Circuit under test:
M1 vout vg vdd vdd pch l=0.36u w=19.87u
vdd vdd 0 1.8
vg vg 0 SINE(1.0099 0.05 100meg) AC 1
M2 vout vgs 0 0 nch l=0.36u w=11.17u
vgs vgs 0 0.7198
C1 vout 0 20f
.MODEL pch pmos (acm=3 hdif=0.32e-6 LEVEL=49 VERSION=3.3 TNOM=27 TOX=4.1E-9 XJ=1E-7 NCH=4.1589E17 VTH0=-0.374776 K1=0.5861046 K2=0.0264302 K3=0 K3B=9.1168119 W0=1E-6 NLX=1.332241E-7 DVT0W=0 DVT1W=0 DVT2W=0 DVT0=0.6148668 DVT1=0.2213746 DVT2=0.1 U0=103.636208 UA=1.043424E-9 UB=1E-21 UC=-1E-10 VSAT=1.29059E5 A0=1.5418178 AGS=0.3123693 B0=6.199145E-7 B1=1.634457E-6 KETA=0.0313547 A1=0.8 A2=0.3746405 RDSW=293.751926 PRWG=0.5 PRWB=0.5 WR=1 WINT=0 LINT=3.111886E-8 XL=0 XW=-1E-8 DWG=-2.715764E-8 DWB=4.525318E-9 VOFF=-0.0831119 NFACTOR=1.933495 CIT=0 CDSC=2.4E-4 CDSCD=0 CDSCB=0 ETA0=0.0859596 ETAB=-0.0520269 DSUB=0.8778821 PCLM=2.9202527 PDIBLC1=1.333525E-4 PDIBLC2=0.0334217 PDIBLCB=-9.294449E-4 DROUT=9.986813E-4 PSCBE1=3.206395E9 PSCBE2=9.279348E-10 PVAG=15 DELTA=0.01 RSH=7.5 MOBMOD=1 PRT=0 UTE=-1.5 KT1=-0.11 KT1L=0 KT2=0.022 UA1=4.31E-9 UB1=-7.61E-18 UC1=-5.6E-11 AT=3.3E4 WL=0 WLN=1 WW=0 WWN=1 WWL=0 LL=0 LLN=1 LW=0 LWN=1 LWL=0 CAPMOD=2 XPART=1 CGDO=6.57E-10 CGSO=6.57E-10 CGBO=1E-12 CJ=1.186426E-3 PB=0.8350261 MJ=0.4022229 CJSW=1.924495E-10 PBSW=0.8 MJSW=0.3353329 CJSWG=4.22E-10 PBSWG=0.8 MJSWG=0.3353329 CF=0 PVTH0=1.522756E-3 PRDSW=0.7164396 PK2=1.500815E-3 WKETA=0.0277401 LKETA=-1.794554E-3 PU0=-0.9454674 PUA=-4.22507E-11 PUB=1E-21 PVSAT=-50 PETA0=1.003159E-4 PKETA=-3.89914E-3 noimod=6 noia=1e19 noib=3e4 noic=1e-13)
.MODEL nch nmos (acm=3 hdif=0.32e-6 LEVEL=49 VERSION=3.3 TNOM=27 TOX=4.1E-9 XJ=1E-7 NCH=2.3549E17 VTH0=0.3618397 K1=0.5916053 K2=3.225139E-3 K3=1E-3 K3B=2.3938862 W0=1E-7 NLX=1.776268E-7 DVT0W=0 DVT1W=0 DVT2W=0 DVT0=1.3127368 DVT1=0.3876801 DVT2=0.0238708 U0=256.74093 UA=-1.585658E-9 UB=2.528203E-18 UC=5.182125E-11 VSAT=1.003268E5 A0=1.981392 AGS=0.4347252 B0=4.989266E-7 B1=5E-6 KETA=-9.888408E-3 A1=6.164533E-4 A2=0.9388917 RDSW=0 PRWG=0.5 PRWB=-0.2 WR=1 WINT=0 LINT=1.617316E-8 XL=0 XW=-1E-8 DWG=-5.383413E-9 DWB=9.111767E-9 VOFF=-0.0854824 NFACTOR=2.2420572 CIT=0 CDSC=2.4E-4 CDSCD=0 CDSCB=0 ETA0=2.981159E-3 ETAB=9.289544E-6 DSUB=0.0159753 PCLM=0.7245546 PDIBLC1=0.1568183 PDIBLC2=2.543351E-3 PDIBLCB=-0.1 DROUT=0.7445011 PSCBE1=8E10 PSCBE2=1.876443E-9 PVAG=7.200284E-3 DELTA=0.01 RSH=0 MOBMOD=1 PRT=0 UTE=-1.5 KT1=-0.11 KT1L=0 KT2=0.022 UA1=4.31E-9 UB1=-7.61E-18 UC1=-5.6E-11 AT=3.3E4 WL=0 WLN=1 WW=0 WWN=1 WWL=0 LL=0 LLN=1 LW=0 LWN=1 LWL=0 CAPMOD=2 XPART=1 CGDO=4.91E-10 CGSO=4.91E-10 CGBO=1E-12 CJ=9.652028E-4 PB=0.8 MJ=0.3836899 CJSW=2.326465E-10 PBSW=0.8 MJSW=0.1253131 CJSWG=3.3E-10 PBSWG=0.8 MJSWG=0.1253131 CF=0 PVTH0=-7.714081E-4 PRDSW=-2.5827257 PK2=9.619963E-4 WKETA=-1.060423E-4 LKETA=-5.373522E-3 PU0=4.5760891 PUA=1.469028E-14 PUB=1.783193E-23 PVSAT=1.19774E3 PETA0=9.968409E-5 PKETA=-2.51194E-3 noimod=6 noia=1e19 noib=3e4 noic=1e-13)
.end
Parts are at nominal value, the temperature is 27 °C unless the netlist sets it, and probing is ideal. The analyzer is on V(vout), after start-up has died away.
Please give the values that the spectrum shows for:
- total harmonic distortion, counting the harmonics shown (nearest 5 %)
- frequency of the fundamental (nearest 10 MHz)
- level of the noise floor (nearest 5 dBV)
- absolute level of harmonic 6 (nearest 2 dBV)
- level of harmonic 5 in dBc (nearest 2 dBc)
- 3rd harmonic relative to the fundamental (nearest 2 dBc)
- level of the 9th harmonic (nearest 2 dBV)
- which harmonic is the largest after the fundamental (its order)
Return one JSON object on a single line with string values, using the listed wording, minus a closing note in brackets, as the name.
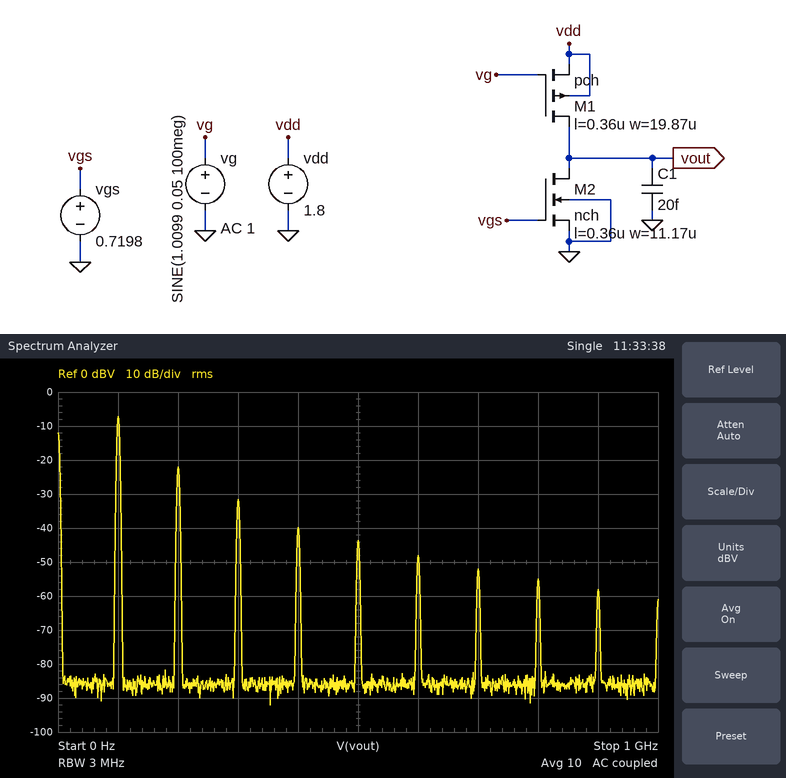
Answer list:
{"total harmonic distortion, counting the harmonics shown": "20 %", "frequency of the fundamental": "100 MHz", "level of the noise floor": "-85 dBV", "absolute level of harmonic 6": "-48 dBV", "level of harmonic 5 in dBc": "-36 dBc", "3rd harmonic relative to the fundamental": "-24 dBc", "level of the 9th harmonic": "-58 dBV", "which harmonic is the largest after the fundamental": "2"}
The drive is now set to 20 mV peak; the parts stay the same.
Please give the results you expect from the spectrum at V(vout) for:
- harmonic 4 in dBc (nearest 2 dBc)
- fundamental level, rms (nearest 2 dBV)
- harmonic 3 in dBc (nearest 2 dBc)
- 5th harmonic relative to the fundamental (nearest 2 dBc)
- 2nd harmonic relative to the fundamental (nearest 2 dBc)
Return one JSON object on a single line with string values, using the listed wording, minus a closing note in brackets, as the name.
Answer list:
{"harmonic 4 in dBc": "-40 dBc", "fundamental level, rms": "-14 dBV", "harmonic 3 in dBc": "-30 dBc", "5th harmonic relative to the fundamental": "-48 dBc", "2nd harmonic relative to the fundamental": "-20 dBc"}
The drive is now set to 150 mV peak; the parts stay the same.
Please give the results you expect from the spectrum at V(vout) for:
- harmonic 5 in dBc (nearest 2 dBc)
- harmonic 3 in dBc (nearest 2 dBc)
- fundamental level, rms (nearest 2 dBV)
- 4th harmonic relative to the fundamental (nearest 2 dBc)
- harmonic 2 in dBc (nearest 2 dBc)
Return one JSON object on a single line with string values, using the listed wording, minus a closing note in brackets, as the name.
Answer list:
{"harmonic 5 in dBc": "-24 dBc", "harmonic 3 in dBc": "-14 dBc", "fundamental level, rms": "-4 dBV", "4th harmonic relative to the fundamental": "-26 dBc", "harmonic 2 in dBc": "-20 dBc"}
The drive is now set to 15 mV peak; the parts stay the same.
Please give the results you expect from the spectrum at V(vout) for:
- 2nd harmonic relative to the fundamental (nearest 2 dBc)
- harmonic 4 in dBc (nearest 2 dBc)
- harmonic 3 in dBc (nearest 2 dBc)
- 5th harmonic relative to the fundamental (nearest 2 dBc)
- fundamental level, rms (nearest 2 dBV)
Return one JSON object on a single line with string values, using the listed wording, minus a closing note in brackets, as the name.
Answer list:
{"2nd harmonic relative to the fundamental": "-22 dBc", "harmonic 4 in dBc": "-46 dBc", "harmonic 3 in dBc": "-34 dBc", "5th harmonic relative to the fundamental": "-56 dBc", "fundamental level, rms": "-16 dBV"}
